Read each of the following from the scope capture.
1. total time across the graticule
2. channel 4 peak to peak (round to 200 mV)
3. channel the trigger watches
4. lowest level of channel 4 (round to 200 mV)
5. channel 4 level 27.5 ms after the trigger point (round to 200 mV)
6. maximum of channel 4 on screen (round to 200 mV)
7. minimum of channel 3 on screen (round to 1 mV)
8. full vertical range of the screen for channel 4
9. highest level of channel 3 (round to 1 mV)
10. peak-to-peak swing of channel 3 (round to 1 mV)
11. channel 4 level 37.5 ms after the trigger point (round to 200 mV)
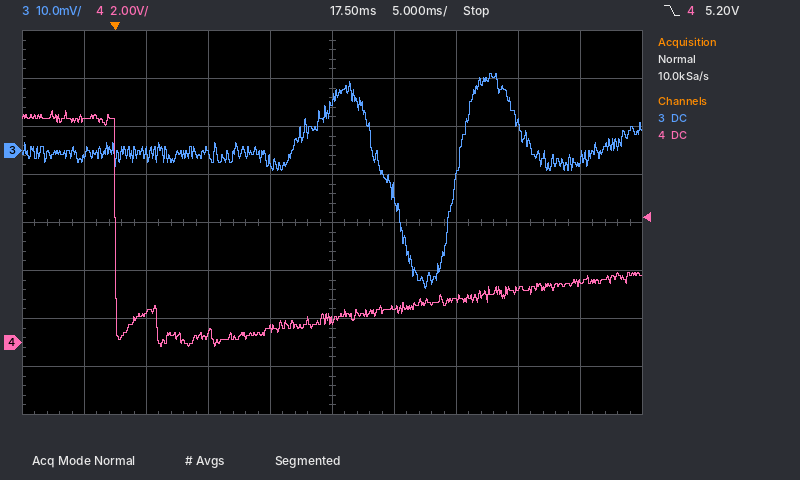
50 ms
9.8 V
channel 4
-200 mV
1.8 V
9.6 V
-29 mV
16 V
16 mV
45 mV
2.4 V
